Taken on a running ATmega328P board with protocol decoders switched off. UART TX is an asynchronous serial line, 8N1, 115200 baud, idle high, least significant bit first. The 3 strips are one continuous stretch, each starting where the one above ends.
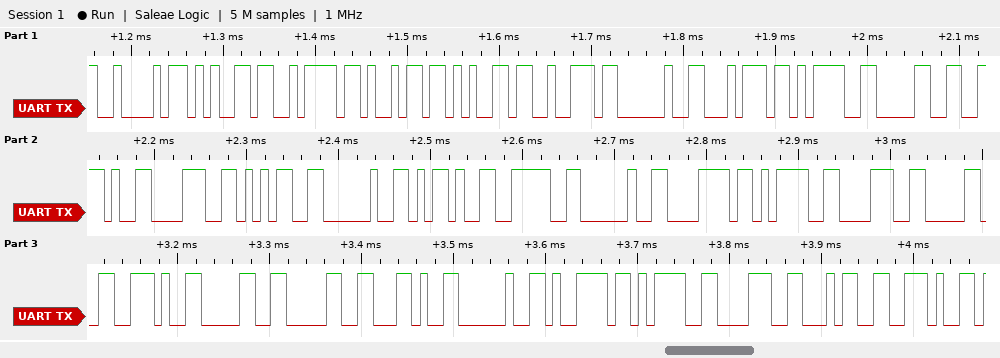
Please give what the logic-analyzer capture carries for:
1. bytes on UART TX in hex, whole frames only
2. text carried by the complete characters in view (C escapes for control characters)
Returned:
42 65 7A 69 65 72 20 74 3D 30 2E 38 35 20 2D 3E 20 78 3D 38 30 2E 30 30 2C 20 79 3D 38 34 2E
"Bezier t=0.85 -> x=80.00, y=84."
